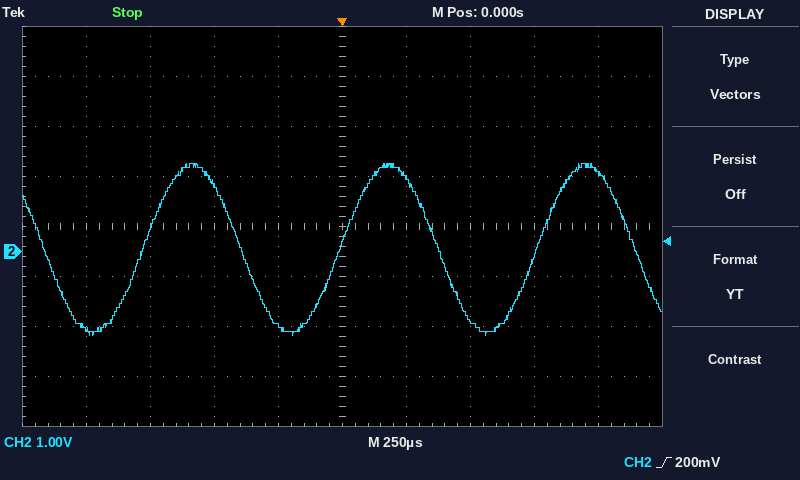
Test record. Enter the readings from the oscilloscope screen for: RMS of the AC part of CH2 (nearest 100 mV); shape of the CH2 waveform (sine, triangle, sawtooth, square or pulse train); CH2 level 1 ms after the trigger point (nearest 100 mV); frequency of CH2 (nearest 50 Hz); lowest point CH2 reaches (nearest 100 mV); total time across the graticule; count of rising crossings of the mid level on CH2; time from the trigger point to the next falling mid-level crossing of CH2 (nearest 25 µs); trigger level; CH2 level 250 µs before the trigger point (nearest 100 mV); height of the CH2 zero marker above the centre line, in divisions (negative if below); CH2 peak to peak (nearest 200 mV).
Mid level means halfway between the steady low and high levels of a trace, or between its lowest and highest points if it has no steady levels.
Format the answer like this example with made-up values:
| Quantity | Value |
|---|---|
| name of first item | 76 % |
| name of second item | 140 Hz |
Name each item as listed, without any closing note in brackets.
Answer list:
| Quantity | Value |
|---|---|
| RMS of the AC part of CH2 | 1.2 V |
| shape of the CH2 waveform | sine |
| CH2 level 1 ms after the trigger point | 1.6 V |
| frequency of CH2 | 1.30 kHz |
| lowest point CH2 reaches | -1.7 V |
| total time across the graticule | 2.5 ms |
| count of rising crossings of the mid level on CH2 | 3 |
| time from the trigger point to the next falling mid-level crossing of CH2 | 375 µs |
| trigger level | 200 mV |
| CH2 level 250 µs before the trigger point | -1.5 V |
| height of the CH2 zero marker above the centre line, in divisions | -0.5 div |
| CH2 peak to peak | 3.4 V |
